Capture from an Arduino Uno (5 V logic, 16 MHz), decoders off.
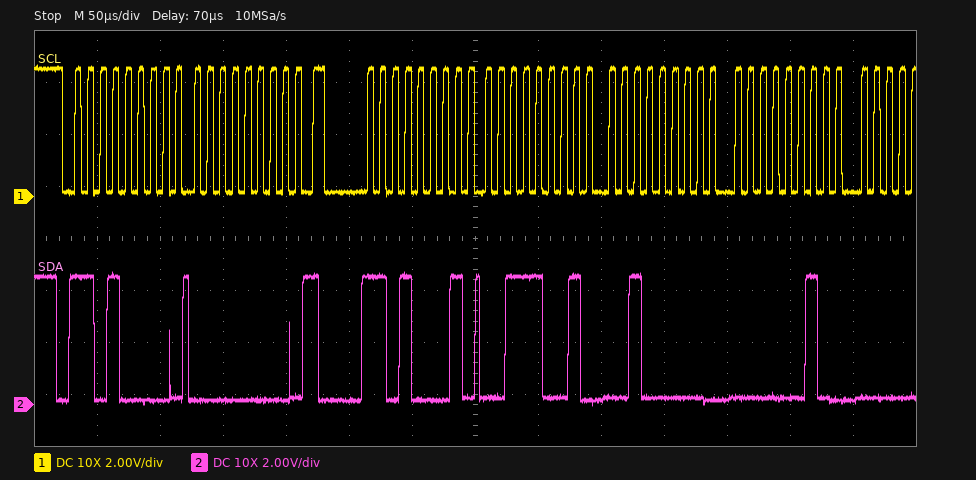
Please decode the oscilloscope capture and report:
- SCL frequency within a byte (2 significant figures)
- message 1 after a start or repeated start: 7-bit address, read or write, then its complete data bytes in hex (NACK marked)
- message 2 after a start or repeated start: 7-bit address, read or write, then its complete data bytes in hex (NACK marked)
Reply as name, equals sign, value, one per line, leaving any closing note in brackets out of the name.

SCL frequency within a byte = 100 kHz
message 1 after a start or repeated start: 7-bit address, read or write, then its complete data bytes in hex = 0x68 write: 00
message 2 after a start or repeated start: 7-bit address, read or write, then its complete data bytes in hex = 0x68 read: 39 20 02
